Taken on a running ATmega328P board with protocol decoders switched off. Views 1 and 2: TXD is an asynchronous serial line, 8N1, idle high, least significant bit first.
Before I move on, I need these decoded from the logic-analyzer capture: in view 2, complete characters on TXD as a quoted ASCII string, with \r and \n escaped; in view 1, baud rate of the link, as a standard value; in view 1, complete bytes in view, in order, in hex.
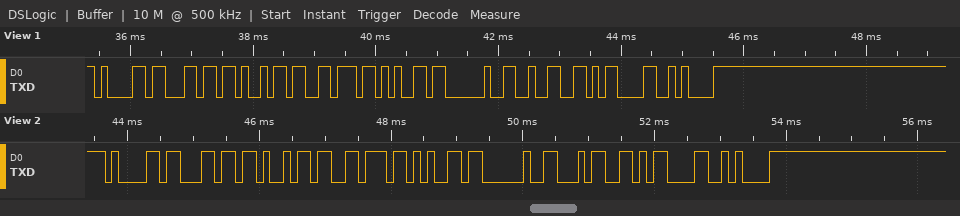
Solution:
"alive 4\r\n"
9600 baud
0x61 0x6C 0x69 0x76 0x65 0x20 0x32 0x0D 0x0A
